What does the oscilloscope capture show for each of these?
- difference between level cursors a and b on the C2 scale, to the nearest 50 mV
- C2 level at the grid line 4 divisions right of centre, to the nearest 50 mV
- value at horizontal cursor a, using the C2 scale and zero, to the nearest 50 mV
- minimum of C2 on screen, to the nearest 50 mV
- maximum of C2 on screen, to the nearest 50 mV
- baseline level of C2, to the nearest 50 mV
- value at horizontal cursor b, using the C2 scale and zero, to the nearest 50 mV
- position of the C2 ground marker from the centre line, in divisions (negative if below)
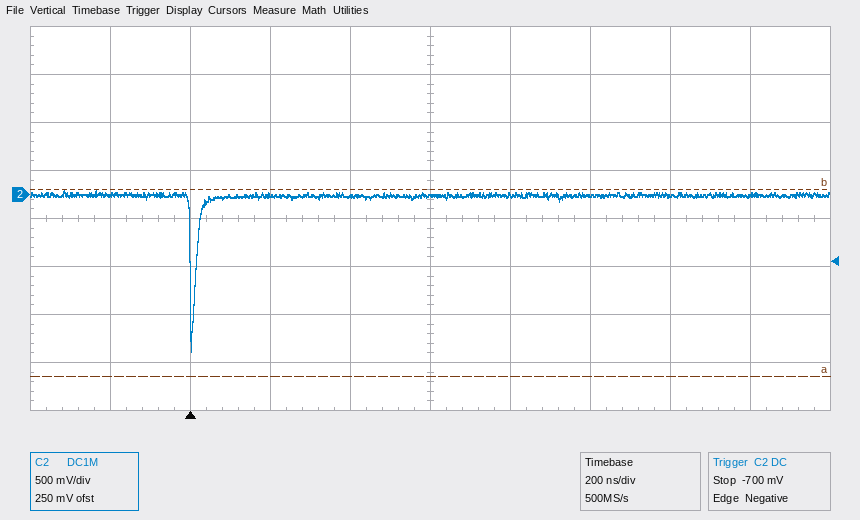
1.95 V
0 mV
-1.90 V
-1.65 V
50 mV
0 mV
50 mV
+0.5 div
